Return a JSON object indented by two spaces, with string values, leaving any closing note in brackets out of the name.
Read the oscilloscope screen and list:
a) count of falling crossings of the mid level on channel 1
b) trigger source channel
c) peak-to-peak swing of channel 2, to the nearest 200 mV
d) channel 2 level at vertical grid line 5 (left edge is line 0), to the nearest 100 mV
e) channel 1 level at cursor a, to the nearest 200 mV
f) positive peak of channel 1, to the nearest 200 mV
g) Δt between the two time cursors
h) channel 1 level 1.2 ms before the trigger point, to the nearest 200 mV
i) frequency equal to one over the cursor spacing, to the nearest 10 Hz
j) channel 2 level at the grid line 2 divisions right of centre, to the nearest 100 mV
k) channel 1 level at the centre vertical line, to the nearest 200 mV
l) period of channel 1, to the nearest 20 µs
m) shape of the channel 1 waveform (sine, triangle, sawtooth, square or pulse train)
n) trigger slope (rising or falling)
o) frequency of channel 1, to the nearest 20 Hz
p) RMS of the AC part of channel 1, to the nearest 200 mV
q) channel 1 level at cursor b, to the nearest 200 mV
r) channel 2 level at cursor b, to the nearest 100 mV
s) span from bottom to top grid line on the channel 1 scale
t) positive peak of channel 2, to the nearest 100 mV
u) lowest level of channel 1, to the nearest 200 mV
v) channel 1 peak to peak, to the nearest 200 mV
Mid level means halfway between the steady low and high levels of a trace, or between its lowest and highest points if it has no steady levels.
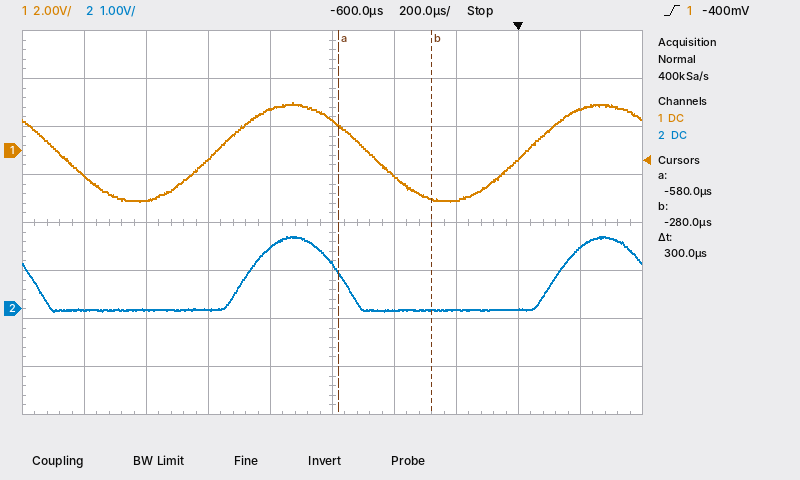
{
  "count of falling crossings of the mid level on channel 1": "2",
  "trigger source channel": "channel 1",
  "peak-to-peak swing of channel 2, to the nearest 200 mV": "1.6 V",
  "channel 2 level at vertical grid line 5 (left edge is line 0), to the nearest 100 mV": "900 mV",
  "channel 1 level at cursor a, to the nearest 200 mV": "1.0 V",
  "positive peak of channel 1, to the nearest 200 mV": "2.0 V",
  "Δt between the two time cursors": "300 µs",
  "channel 1 level 1.2 ms before the trigger point, to the nearest 200 mV": "-2.0 V",
  "frequency equal to one over the cursor spacing, to the nearest 10 Hz": "3.33 kHz",
  "channel 2 level at the grid line 2 divisions right of centre, to the nearest 100 mV": "0.0 V",
  "channel 1 level at the centre vertical line, to the nearest 200 mV": "1.2 V",
  "period of channel 1, to the nearest 20 µs": "1.00 ms",
  "shape of the channel 1 waveform": "sine",
  "trigger slope": "rising",
  "frequency of channel 1, to the nearest 20 Hz": "1.00 kHz",
  "RMS of the AC part of channel 1, to the nearest 200 mV": "1.4 V",
  "channel 1 level at cursor b, to the nearest 200 mV": "-2.0 V",
  "channel 2 level at cursor b, to the nearest 100 mV": "0.0 V",
  "span from bottom to top grid line on the channel 1 scale": "16 V",
  "positive peak of channel 2, to the nearest 100 mV": "1.5 V",
  "lowest level of channel 1, to the nearest 200 mV": "-2.2 V",
  "channel 1 peak to peak, to the nearest 200 mV": "4.2 V"
}
